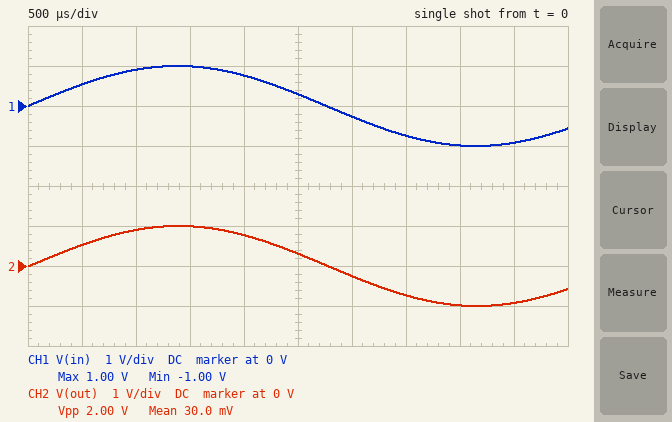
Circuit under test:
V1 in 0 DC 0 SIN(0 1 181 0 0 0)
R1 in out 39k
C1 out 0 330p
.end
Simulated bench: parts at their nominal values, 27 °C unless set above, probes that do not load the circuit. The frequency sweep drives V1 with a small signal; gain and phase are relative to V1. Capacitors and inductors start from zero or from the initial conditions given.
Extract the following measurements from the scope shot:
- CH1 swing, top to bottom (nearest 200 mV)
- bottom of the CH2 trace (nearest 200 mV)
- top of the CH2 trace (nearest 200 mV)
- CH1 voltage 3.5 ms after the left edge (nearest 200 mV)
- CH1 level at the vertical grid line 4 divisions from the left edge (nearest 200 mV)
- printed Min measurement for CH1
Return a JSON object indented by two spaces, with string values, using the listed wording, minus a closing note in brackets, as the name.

{
  "CH1 swing, top to bottom": "2.0 V",
  "bottom of the CH2 trace": "-1.0 V",
  "top of the CH2 trace": "1.0 V",
  "CH1 voltage 3.5 ms after the left edge": "-800 mV",
  "CH1 level at the vertical grid line 4 divisions from the left edge": "800 mV",
  "printed Min measurement for CH1": "-1.00 V"
}
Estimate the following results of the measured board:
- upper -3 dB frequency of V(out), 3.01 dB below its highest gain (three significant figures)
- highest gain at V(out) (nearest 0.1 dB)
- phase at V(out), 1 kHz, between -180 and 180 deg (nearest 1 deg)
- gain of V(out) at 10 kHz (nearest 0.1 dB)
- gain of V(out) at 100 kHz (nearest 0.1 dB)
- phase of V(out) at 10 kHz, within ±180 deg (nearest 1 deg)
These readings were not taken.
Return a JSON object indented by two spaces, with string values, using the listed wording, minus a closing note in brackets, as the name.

{
  "upper -3 dB frequency of V(out), 3.01 dB below its highest gain": "12.4 kHz",
  "highest gain at V(out)": "0 dB",
  "phase at V(out), 1 kHz, between -180 and 180 deg": "-5 deg",
  "gain of V(out) at 10 kHz": "-2.2 dB",
  "gain of V(out) at 100 kHz": "-18.2 dB",
  "phase of V(out) at 10 kHz, within ±180 deg": "-39 deg"
}
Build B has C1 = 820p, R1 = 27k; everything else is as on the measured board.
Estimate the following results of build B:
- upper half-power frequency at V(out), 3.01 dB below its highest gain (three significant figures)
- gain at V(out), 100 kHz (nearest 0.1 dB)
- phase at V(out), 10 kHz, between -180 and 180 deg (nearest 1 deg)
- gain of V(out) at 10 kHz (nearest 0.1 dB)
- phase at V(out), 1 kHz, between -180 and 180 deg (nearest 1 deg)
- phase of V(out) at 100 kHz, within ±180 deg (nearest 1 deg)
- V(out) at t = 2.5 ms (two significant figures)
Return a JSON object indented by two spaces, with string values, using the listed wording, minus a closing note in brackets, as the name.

{
  "upper half-power frequency at V(out), 3.01 dB below its highest gain": "7.19 kHz",
  "gain at V(out), 100 kHz": "-22.9 dB",
  "phase at V(out), 10 kHz, between -180 and 180 deg": "-54 deg",
  "gain of V(out) at 10 kHz": "-4.7 dB",
  "phase at V(out), 1 kHz, between -180 and 180 deg": "-8 deg",
  "phase of V(out) at 100 kHz, within ±180 deg": "-86 deg",
  "V(out) at t = 2.5 ms": "320 mV"
}
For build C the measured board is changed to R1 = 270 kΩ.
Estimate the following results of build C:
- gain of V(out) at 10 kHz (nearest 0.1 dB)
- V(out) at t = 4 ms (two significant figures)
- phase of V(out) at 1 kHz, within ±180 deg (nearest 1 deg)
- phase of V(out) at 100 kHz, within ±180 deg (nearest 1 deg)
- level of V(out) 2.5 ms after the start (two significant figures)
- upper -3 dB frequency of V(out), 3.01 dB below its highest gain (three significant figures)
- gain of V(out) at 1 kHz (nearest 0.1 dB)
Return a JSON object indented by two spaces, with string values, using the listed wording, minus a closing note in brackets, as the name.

{
  "gain of V(out) at 10 kHz": "-15.1 dB",
  "V(out) at t = 4 ms": "-960 mV",
  "phase of V(out) at 1 kHz, within ±180 deg": "-29 deg",
  "phase of V(out) at 100 kHz, within ±180 deg": "-89 deg",
  "level of V(out) 2.5 ms after the start": "390 mV",
  "upper -3 dB frequency of V(out), 3.01 dB below its highest gain": "1.79 kHz",
  "gain of V(out) at 1 kHz": "-1.2 dB"
}
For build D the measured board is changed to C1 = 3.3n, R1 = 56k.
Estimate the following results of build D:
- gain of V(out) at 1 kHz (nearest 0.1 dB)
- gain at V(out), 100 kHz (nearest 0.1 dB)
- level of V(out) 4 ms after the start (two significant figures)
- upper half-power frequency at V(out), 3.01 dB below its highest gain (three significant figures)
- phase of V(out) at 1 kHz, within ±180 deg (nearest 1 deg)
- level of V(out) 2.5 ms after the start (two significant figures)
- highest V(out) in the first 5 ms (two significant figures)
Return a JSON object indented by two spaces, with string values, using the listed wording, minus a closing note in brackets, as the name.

{
  "gain of V(out) at 1 kHz": "-3.7 dB",
  "gain at V(out), 100 kHz": "-41.3 dB",
  "level of V(out) 4 ms after the start": "-910 mV",
  "upper half-power frequency at V(out), 3.01 dB below its highest gain": "861 Hz",
  "phase of V(out) at 1 kHz, within ±180 deg": "-49 deg",
  "level of V(out) 2.5 ms after the start": "470 mV",
  "highest V(out) in the first 5 ms": "980 mV"
}
